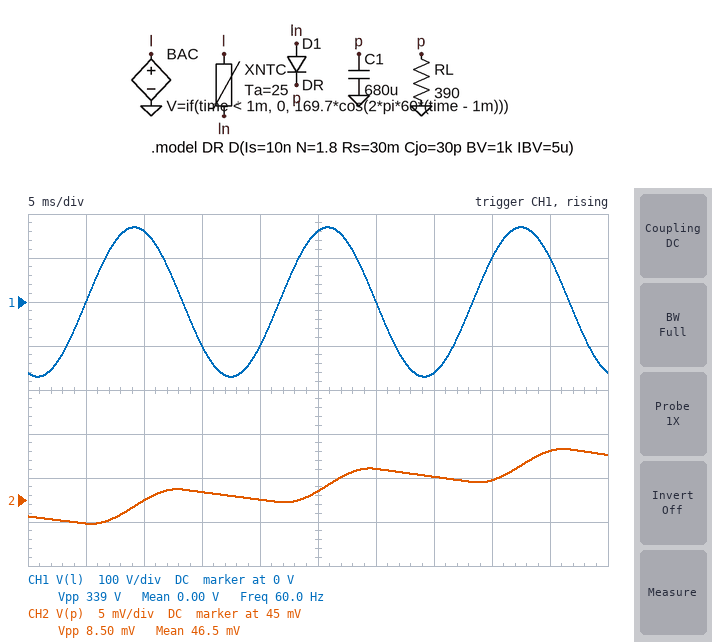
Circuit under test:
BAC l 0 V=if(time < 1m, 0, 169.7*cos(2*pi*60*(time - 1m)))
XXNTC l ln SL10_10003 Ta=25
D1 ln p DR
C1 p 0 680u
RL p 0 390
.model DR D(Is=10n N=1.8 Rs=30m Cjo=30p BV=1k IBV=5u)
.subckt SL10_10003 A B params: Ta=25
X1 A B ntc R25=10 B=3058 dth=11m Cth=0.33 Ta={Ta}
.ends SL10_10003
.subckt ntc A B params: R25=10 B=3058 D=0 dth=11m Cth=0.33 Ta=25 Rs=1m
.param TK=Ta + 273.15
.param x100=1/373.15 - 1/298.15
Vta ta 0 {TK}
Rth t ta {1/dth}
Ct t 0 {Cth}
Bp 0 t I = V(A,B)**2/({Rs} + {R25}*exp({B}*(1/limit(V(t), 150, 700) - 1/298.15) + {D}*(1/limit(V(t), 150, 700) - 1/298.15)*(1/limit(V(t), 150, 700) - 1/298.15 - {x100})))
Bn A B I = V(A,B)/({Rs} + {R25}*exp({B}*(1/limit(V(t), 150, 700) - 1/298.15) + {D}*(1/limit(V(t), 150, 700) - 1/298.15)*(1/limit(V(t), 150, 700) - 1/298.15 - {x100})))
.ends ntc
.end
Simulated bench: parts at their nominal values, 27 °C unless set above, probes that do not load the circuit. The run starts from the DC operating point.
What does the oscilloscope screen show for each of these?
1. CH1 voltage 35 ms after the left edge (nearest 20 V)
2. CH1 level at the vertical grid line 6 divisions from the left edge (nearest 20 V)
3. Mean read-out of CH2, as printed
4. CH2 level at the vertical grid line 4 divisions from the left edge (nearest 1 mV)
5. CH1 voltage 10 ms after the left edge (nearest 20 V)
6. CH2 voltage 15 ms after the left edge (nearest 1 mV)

-160 V
0 V
46.5 mV
45 mV
160 V
46 mV
